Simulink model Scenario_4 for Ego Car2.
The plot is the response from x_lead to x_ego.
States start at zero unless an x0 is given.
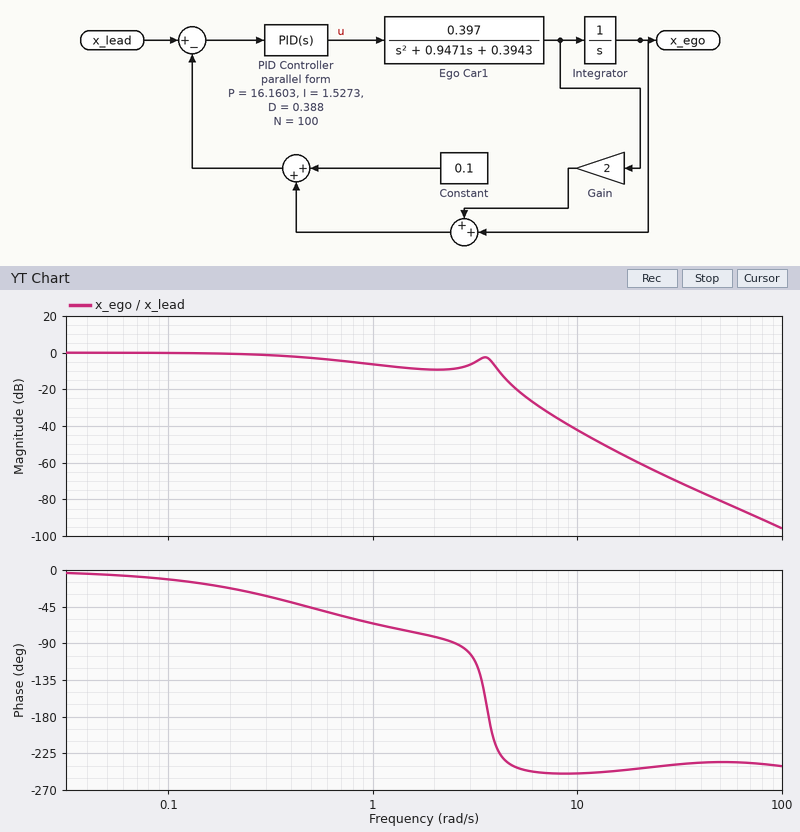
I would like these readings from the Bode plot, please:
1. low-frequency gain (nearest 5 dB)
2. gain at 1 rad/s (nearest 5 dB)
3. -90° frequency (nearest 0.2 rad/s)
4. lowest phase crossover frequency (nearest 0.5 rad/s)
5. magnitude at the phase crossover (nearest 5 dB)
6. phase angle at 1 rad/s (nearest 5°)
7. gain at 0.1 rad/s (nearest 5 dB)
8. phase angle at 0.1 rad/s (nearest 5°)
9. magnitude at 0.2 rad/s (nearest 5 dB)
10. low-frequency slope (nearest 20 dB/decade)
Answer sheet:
0 dB
-5 dB
2.6 rad/s
3.5 rad/s
-5 dB
-65°
0 dB
-10°
0 dB
0 dB/decade
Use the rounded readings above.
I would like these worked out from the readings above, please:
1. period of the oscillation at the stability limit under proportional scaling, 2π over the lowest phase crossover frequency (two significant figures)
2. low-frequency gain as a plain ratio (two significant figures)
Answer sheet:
1.8 s
1.0
